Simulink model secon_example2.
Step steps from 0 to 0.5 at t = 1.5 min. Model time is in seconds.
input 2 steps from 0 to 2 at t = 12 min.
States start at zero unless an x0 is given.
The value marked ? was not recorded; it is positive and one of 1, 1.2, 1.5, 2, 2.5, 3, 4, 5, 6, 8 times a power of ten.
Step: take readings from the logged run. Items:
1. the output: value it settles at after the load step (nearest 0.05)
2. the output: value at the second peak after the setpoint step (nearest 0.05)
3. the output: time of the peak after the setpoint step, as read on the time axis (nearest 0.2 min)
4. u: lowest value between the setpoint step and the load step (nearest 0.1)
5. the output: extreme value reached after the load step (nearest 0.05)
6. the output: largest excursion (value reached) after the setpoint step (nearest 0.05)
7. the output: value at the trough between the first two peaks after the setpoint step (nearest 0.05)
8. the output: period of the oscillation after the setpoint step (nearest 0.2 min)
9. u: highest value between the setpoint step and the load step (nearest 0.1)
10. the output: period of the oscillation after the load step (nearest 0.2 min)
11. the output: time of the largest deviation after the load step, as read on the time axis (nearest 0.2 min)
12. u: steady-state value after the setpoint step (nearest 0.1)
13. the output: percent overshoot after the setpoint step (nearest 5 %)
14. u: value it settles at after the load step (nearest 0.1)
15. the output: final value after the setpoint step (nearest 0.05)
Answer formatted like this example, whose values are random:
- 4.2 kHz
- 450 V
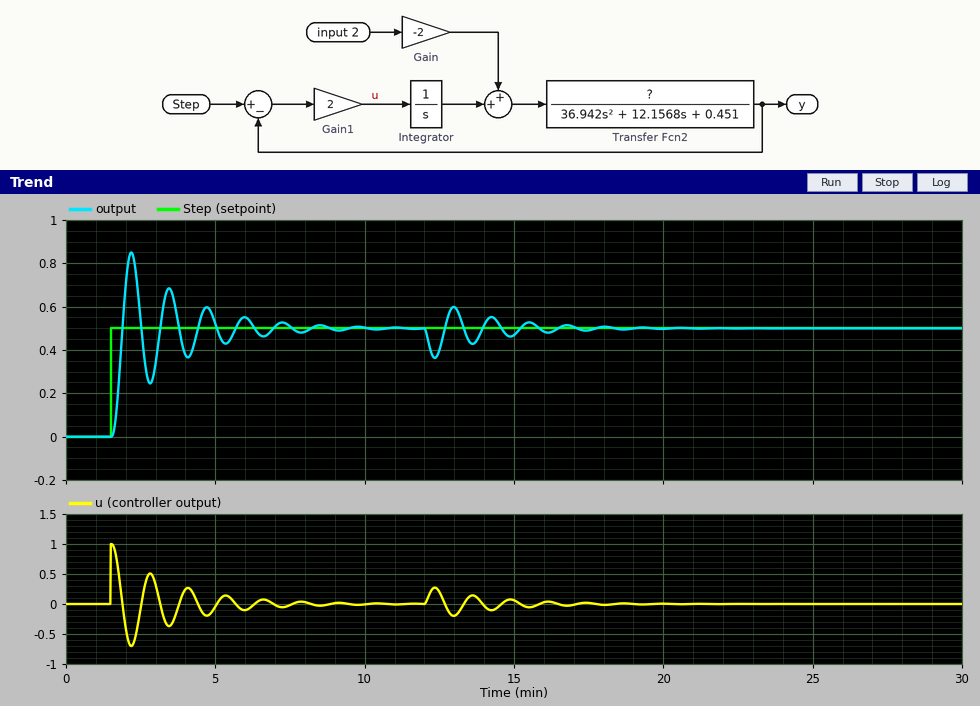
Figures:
- 0.50
- 0.70
- 2.2 min
- -0.7
- 0.35
- 0.85
- 0.25
- 1.2 min
- 1.0
- 1.2 min
- 12.4 min
- 0.0
- 70 %
- 0.0
- 0.50
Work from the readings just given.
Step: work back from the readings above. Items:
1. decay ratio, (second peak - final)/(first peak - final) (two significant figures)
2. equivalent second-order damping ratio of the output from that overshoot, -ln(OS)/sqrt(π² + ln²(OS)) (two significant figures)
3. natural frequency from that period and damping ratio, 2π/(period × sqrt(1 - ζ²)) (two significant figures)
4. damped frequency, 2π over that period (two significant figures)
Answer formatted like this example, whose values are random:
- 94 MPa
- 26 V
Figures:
- 0.57
- 0.11
- 5.3 rad/min
- 5.2 rad/min
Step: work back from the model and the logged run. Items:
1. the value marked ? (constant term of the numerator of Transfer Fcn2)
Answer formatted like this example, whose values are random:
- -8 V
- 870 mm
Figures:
- 0.04
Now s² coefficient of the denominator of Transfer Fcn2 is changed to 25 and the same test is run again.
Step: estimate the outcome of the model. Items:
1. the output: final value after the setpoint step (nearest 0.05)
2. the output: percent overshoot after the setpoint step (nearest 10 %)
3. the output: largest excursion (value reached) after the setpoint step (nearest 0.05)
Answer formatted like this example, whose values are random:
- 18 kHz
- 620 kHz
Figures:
- 0.50
- 60 %
- 0.80
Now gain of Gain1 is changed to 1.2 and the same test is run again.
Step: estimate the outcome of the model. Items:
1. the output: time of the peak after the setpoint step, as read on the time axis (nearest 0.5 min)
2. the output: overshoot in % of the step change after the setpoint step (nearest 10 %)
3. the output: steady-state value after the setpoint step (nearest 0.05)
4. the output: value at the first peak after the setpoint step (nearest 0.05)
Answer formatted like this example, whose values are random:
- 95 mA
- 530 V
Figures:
- 2.5 min
- 50 %
- 0.50
- 0.75
